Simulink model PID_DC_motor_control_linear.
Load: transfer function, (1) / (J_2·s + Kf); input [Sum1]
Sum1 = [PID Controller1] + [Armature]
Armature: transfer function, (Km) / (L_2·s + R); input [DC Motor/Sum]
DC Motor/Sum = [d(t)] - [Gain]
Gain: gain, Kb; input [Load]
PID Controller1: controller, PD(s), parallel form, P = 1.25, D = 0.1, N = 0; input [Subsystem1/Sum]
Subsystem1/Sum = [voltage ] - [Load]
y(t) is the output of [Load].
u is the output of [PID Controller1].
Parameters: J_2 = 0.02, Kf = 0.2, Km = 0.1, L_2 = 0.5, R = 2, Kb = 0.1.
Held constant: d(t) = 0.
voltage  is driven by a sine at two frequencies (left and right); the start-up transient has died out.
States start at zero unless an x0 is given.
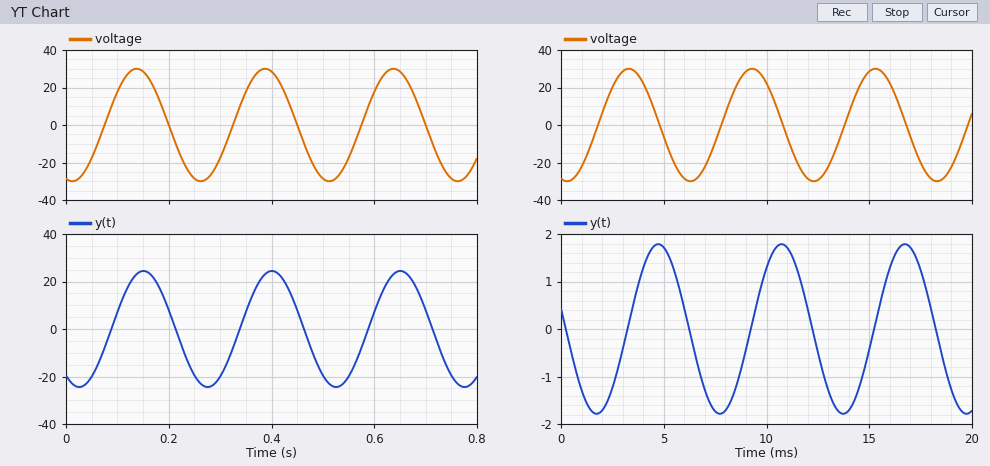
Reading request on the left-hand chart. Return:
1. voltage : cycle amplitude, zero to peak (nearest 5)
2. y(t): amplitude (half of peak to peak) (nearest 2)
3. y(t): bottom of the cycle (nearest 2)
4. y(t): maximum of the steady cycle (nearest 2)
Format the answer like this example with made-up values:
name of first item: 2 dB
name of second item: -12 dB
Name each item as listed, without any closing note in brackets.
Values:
voltage : cycle amplitude, zero to peak: 30
y(t): amplitude (half of peak to peak): 24
y(t): bottom of the cycle: -24
y(t): maximum of the steady cycle: 24
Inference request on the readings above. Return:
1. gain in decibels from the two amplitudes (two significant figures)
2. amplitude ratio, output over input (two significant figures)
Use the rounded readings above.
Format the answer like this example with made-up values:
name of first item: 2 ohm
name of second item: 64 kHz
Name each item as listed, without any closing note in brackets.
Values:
gain in decibels from the two amplitudes: -1.9 dB
amplitude ratio, output over input: 0.80
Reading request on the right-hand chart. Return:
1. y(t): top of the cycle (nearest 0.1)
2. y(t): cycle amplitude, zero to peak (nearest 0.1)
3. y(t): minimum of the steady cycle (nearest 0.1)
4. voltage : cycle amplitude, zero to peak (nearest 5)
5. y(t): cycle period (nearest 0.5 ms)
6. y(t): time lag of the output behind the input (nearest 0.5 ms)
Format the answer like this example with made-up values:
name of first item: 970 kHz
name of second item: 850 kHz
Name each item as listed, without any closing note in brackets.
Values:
y(t): top of the cycle: 1.8
y(t): cycle amplitude, zero to peak: 1.8
y(t): minimum of the steady cycle: -1.8
voltage : cycle amplitude, zero to peak: 30
y(t): cycle period: 6.0 ms
y(t): time lag of the output behind the input: 1.5 ms
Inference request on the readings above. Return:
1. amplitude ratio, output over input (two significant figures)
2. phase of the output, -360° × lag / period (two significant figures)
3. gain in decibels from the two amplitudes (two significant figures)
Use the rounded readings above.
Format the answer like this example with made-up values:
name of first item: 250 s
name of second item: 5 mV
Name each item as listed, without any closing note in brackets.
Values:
amplitude ratio, output over input: 0.060
phase of the output, -360° × lag / period: -90°
gain in decibels from the two amplitudes: -24 dB
